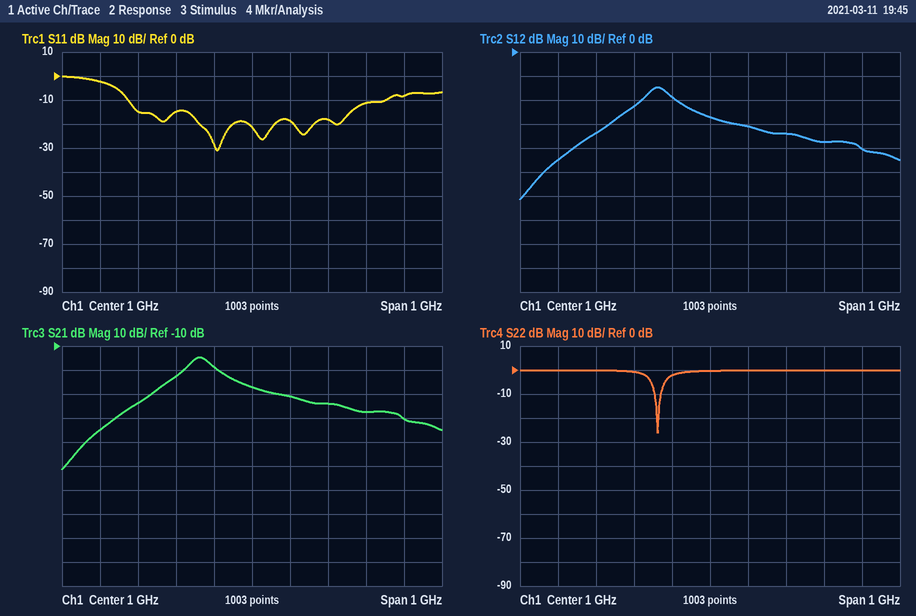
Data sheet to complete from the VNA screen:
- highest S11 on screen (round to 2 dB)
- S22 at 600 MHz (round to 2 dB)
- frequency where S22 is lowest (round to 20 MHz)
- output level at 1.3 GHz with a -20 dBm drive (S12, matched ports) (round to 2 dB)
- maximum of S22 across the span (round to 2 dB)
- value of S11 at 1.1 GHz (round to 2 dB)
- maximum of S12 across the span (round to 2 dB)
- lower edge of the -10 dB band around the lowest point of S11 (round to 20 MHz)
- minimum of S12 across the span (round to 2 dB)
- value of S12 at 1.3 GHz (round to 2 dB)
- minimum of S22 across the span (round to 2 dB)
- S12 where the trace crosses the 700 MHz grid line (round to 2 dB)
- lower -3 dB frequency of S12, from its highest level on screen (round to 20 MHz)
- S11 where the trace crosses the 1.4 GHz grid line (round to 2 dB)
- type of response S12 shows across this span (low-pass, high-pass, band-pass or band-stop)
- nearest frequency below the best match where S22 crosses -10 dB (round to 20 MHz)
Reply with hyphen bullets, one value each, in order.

- 0 dB
- 0 dB
- 860 MHz
- -58 dBm
- 0 dB
- -18 dB
- -14 dB
- 680 MHz
- -62 dB
- -38 dB
- -26 dB
- -34 dB
- 840 MHz
- -8 dB
- band-pass
- 860 MHz
